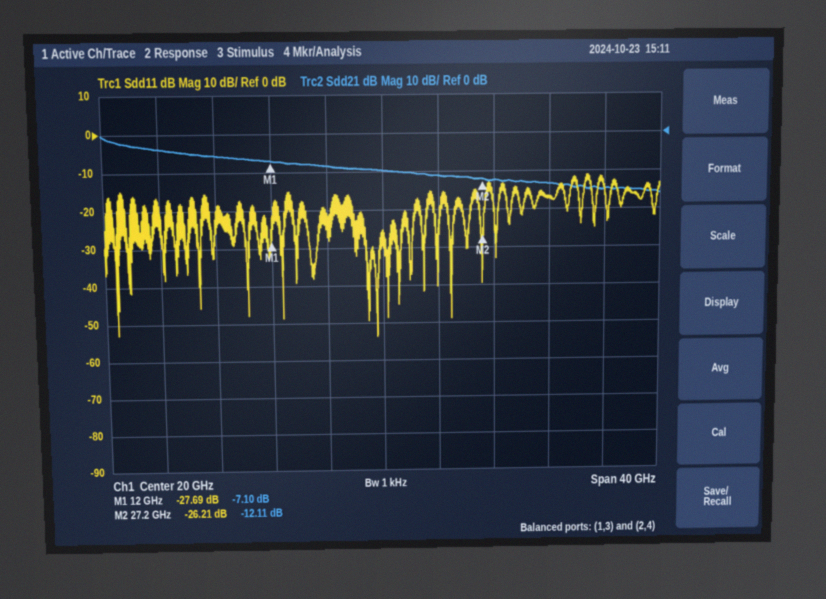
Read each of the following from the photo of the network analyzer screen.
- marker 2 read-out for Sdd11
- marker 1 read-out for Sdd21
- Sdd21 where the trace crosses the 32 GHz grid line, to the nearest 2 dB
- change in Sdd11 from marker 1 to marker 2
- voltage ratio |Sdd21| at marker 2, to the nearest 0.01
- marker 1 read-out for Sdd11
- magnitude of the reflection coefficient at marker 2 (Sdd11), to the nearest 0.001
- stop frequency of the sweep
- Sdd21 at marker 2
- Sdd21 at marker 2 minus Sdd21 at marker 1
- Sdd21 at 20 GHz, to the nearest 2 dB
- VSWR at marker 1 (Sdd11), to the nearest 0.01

-26.21 dB
-7.10 dB
-14 dB
1.48 dB
0.25
-27.69 dB
0.049
40 GHz
-12.11 dB
-5.01 dB
-10 dB
1.09
